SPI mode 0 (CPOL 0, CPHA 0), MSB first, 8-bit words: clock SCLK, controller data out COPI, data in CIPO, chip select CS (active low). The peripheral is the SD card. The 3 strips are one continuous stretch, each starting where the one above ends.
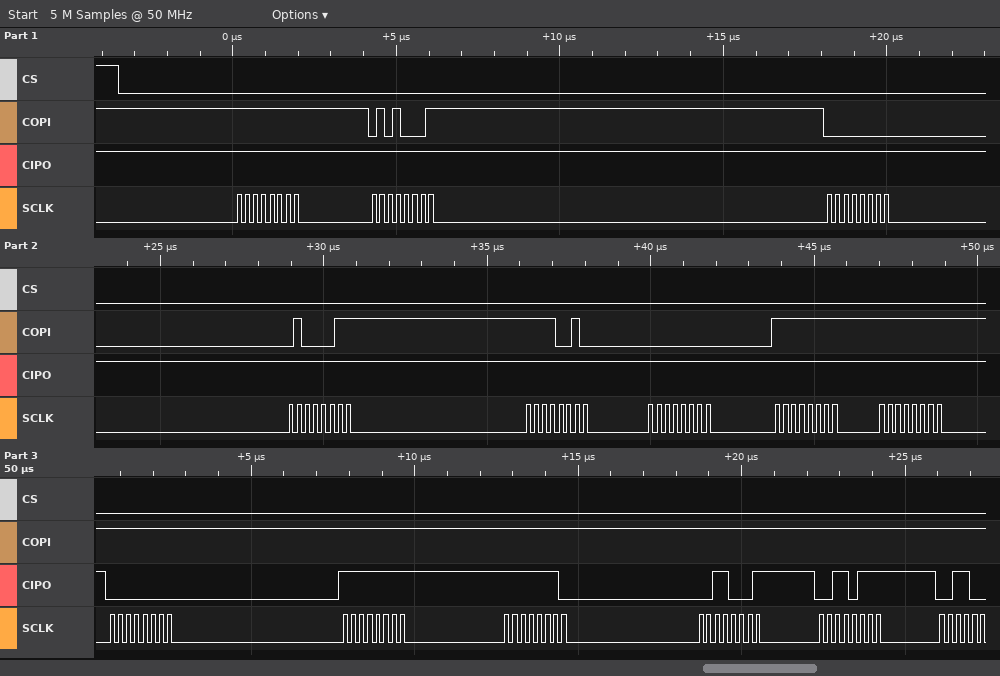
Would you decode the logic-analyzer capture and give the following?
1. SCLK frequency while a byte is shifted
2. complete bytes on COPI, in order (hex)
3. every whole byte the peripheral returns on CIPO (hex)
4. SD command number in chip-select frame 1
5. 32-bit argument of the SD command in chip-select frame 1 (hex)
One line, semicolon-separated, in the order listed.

4 MHz; 0xFF 0x51 0x00 0x43 0xF2 0x00 0xFF 0xFF 0xFF 0xFF 0xFF 0xFF 0xFF; 0xFF 0xFF 0xFF 0xFF 0xFF 0xFF 0xFF 0xFF 0x00 0xFF 0xFE 0x31 0x37; CMD17; 0x0043F200
